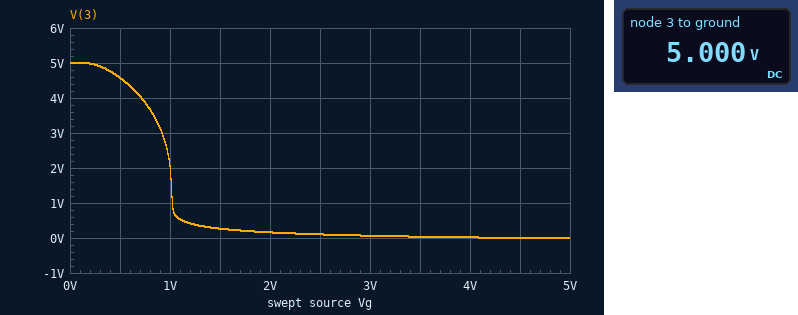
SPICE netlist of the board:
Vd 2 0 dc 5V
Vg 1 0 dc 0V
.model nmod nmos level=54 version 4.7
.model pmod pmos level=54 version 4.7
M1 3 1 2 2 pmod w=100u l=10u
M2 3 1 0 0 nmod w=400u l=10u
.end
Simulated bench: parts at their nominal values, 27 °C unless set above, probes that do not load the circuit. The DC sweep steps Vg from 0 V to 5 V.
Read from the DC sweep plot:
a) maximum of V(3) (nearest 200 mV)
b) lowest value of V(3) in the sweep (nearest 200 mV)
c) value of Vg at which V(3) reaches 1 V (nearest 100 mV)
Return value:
5.0 V
0 V
1.0 V
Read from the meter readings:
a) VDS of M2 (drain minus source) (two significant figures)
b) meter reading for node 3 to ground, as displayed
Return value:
5.0 V
5.000 V
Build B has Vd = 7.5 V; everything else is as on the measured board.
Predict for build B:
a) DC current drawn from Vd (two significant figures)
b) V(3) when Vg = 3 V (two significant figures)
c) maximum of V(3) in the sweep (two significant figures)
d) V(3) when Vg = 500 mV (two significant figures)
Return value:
480 nA
240 mV
7.5 V
6.9 V
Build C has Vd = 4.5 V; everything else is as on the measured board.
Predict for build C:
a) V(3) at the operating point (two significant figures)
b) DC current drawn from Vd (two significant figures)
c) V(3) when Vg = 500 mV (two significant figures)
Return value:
4.5 V
200 nA
4.1 V
